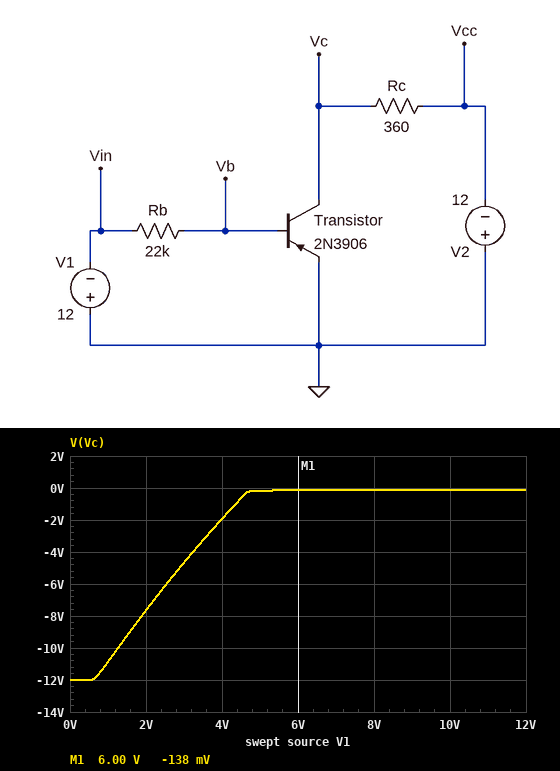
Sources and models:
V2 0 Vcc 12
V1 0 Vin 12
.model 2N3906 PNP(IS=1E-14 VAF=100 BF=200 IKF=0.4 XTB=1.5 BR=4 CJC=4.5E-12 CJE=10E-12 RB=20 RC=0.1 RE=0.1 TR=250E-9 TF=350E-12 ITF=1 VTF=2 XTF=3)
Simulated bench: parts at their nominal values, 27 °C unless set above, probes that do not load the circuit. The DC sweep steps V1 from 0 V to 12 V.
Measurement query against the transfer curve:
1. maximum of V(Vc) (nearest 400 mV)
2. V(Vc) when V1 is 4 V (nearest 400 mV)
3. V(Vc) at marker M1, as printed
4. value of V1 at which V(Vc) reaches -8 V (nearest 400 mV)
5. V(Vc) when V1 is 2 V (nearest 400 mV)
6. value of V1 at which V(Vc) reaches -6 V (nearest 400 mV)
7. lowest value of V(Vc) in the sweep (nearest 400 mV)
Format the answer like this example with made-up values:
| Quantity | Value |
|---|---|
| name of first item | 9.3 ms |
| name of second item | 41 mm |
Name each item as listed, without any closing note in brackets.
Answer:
| Quantity | Value |
|---|---|
| maximum of V(Vc) | 0 V |
| V(Vc) when V1 is 4 V | -2.0 V |
| V(Vc) at marker M1, as printed | -138 mV |
| value of V1 at which V(Vc) reaches -8 V | 2.0 V |
| V(Vc) when V1 is 2 V | -7.6 V |
| value of V1 at which V(Vc) reaches -6 V | 2.4 V |
| lowest value of V(Vc) in the sweep | -12.0 V |
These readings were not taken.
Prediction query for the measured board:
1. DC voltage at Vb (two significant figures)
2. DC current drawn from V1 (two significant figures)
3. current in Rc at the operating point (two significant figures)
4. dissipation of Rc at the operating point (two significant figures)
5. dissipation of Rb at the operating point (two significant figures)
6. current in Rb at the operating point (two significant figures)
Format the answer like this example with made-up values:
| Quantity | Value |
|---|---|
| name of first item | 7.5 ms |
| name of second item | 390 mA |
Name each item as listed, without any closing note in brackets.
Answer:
| Quantity | Value |
|---|---|
| DC voltage at Vb | -760 mV |
| DC current drawn from V1 | 510 µA |
| current in Rc at the operating point | 33 mA |
| dissipation of Rc at the operating point | 390 mW |
| dissipation of Rb at the operating point | 5.7 mW |
| current in Rb at the operating point | 510 µA |
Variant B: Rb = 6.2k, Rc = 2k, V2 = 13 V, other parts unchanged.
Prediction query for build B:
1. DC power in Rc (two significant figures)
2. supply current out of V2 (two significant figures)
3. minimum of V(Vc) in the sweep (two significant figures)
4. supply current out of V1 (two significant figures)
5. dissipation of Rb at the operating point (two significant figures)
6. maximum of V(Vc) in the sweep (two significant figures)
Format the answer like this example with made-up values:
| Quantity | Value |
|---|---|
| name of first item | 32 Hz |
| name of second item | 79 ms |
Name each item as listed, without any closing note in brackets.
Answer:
| Quantity | Value |
|---|---|
| DC power in Rc | 84 mW |
| supply current out of V2 | 6.5 mA |
| minimum of V(Vc) in the sweep | -13 V |
| supply current out of V1 | 1.8 mA |
| dissipation of Rb at the operating point | 20 mW |
| maximum of V(Vc) in the sweep | -22 mV |
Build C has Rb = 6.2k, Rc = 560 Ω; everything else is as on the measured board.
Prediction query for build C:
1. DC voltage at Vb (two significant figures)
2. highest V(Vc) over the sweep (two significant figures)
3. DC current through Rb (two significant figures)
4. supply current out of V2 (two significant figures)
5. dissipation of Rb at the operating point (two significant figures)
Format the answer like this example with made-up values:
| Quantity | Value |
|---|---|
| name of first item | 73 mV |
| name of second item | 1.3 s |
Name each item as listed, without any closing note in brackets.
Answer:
| Quantity | Value |
|---|---|
| DC voltage at Vb | -780 mV |
| highest V(Vc) over the sweep | -45 mV |
| DC current through Rb | 1.8 mA |
| supply current out of V2 | 21 mA |
| dissipation of Rb at the operating point | 20 mW |
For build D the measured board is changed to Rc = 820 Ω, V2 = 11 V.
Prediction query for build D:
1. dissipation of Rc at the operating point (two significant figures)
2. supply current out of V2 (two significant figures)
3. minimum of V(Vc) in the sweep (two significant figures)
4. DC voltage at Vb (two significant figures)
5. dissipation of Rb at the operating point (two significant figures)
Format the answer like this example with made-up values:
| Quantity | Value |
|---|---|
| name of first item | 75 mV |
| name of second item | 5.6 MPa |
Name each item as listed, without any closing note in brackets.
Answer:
| Quantity | Value |
|---|---|
| dissipation of Rc at the operating point | 150 mW |
| supply current out of V2 | 13 mA |
| minimum of V(Vc) in the sweep | -11 V |
| DC voltage at Vb | -740 mV |
| dissipation of Rb at the operating point | 5.8 mW |
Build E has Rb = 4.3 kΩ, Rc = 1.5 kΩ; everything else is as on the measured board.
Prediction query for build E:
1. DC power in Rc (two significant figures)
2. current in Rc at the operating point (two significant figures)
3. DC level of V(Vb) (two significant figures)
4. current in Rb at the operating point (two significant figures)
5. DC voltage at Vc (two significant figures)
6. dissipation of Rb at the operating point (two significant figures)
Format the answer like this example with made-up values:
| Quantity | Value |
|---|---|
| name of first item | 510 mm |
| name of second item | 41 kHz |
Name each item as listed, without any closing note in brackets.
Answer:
| Quantity | Value |
|---|---|
| DC power in Rc | 96 mW |
| current in Rc at the operating point | 8.0 mA |
| DC level of V(Vb) | -790 mV |
| current in Rb at the operating point | 2.6 mA |
| DC voltage at Vc | -21 mV |
| dissipation of Rb at the operating point | 29 mW |
